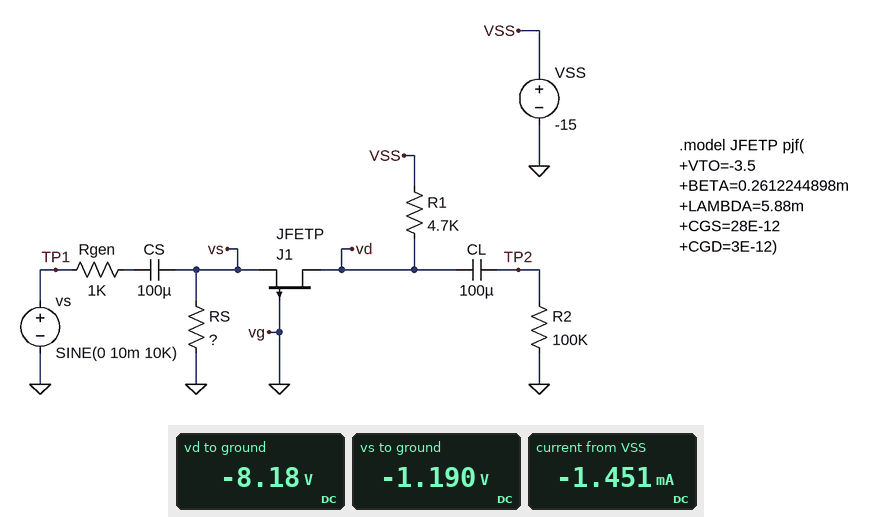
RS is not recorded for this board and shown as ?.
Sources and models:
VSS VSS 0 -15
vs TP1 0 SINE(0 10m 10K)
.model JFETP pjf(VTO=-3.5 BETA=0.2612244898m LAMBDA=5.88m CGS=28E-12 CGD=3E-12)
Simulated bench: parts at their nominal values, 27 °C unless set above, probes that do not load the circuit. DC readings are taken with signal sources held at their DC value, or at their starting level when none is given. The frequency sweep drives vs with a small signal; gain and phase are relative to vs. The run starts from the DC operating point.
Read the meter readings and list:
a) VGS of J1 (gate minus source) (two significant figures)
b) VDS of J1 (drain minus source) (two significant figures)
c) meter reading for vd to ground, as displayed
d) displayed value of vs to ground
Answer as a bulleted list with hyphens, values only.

- 1.2 V
- -7.0 V
- -8.18 V
- -1.190 V
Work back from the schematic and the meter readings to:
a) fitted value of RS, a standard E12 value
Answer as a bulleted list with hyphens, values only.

- 820 Ω
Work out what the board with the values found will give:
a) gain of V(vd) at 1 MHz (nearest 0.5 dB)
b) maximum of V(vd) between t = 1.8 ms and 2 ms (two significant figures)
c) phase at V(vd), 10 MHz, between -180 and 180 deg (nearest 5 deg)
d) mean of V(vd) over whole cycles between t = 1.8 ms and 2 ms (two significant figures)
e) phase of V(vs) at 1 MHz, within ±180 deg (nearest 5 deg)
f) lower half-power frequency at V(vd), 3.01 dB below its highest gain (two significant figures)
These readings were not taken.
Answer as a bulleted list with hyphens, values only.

- 4.0 dB
- -8.2 V
- -35 deg
- -8.2 V
- 0 deg
- 1.1 Hz
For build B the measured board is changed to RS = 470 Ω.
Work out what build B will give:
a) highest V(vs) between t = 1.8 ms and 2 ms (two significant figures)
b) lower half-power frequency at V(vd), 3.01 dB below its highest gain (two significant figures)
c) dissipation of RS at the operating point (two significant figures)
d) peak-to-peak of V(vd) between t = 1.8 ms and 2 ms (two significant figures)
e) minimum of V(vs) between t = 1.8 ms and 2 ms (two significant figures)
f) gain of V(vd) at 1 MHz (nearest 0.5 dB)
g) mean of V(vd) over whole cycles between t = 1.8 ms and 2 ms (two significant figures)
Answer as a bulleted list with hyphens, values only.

- -870 mV
- 1.2 Hz
- 1.6 mW
- 27 mV
- -880 mV
- 2.5 dB
- -6.3 V
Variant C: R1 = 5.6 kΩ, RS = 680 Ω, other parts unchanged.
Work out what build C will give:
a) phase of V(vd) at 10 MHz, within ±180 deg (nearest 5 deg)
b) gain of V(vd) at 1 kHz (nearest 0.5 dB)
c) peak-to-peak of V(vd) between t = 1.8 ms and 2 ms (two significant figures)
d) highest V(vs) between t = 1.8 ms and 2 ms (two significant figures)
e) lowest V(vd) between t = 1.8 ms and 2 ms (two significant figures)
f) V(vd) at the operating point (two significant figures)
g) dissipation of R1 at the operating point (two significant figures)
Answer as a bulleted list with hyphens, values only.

- -40 deg
- 5.0 dB
- 36 mV
- -1.1 V
- -6.2 V
- -6.1 V
- 14 mW
